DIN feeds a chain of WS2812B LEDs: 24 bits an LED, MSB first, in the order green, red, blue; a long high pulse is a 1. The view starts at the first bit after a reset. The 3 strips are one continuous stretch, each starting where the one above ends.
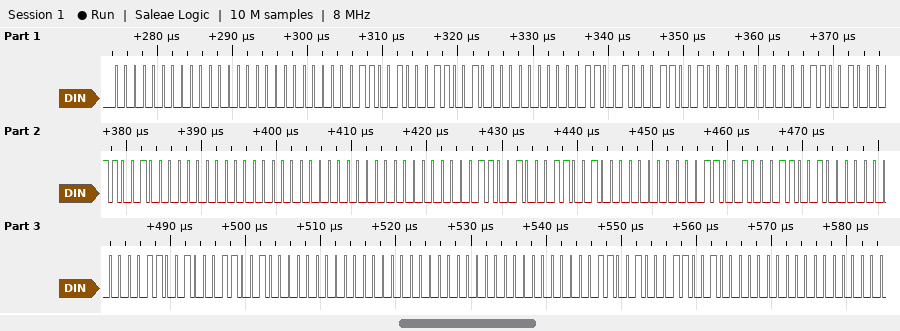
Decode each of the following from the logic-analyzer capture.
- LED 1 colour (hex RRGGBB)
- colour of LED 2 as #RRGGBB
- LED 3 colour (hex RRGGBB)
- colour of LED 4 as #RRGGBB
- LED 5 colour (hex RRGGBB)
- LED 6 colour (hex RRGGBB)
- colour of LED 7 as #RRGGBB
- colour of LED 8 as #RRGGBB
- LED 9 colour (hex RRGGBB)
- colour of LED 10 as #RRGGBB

#000000
#323200
#323200
#323200
#000000
#323200
#323200
#323200
#000000
#323200
